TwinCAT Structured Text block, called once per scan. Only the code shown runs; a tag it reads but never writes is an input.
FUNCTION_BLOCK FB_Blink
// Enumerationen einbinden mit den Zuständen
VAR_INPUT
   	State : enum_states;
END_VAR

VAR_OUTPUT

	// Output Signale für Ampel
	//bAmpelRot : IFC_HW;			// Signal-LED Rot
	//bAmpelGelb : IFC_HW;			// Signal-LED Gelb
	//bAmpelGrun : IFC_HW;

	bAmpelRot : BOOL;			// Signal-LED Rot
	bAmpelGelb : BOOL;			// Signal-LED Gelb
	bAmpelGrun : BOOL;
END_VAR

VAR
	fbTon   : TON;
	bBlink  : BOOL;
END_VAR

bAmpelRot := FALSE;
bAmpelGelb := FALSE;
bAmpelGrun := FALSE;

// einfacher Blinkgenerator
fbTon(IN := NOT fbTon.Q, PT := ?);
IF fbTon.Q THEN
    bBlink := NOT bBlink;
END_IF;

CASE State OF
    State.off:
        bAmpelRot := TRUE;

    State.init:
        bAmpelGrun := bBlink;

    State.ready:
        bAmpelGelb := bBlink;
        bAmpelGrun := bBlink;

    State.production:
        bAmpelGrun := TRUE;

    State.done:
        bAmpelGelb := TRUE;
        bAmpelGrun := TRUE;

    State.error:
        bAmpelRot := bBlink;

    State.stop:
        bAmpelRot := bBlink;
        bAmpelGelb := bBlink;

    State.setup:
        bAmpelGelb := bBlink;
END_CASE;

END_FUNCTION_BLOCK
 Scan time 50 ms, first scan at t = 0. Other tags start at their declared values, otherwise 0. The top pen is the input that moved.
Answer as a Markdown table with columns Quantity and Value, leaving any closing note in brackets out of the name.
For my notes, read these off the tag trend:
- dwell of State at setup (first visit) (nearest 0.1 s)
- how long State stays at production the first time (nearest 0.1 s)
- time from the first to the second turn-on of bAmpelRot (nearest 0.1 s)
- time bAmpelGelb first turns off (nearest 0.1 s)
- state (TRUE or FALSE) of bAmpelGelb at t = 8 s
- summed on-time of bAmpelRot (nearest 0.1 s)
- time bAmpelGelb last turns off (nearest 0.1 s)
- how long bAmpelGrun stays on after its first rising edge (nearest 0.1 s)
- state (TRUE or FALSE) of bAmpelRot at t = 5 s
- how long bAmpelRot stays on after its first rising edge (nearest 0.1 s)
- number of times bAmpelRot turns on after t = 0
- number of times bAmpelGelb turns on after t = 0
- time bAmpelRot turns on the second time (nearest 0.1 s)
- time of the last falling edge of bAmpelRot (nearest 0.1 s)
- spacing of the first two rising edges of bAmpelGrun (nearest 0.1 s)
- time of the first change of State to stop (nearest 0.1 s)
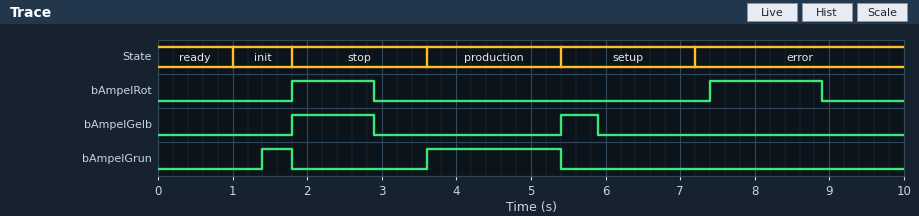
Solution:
| Quantity | Value |
|---|---|
| dwell of State at setup (first visit) | 1.8 s |
| how long State stays at production the first time | 1.8 s |
| time from the first to the second turn-on of bAmpelRot | 5.6 s |
| time bAmpelGelb first turns off | 2.9 s |
| state (TRUE or FALSE) of bAmpelGelb at t = 8 s | FALSE |
| summed on-time of bAmpelRot | 2.6 s |
| time bAmpelGelb last turns off | 5.9 s |
| how long bAmpelGrun stays on after its first rising edge | 0.4 s |
| state (TRUE or FALSE) of bAmpelRot at t = 5 s | FALSE |
| how long bAmpelRot stays on after its first rising edge | 1.1 s |
| number of times bAmpelRot turns on after t = 0 | 2 |
| number of times bAmpelGelb turns on after t = 0 | 2 |
| time bAmpelRot turns on the second time | 7.4 s |
| time of the last falling edge of bAmpelRot | 8.9 s |
| spacing of the first two rising edges of bAmpelGrun | 2.2 s |
| time of the first change of State to stop | 1.8 s |
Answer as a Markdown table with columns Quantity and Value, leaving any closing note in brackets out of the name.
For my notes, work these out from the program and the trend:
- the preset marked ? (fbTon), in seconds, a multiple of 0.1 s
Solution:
| Quantity | Value |
|---|---|
| the preset marked ? (fbTon), in seconds, a multiple of 0.1 s | 1.4 s |
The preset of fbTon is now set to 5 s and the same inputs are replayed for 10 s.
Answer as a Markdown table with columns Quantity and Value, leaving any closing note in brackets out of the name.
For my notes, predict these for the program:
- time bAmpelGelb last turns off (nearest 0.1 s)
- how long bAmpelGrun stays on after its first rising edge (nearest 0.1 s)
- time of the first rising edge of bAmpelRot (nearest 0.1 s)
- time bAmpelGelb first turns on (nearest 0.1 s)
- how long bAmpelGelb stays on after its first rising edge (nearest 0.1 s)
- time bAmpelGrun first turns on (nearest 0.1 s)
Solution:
| Quantity | Value |
|---|---|
| time bAmpelGelb last turns off | 7.2 s |
| how long bAmpelGrun stays on after its first rising edge | 1.8 s |
| time of the first rising edge of bAmpelRot | 7.2 s |
| time bAmpelGelb first turns on | 5.4 s |
| how long bAmpelGelb stays on after its first rising edge | 1.8 s |
| time bAmpelGrun first turns on | 3.6 s |
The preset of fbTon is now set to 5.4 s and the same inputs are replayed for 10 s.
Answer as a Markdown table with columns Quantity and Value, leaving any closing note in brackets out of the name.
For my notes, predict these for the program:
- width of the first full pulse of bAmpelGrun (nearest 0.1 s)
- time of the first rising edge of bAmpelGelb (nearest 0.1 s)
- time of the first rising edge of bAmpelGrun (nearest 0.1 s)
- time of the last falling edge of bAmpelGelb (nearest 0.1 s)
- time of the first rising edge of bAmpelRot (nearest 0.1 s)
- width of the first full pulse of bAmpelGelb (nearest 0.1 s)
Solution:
| Quantity | Value |
|---|---|
| width of the first full pulse of bAmpelGrun | 1.8 s |
| time of the first rising edge of bAmpelGelb | 5.4 s |
| time of the first rising edge of bAmpelGrun | 3.6 s |
| time of the last falling edge of bAmpelGelb | 7.2 s |
| time of the first rising edge of bAmpelRot | 7.2 s |
| width of the first full pulse of bAmpelGelb | 1.8 s |
